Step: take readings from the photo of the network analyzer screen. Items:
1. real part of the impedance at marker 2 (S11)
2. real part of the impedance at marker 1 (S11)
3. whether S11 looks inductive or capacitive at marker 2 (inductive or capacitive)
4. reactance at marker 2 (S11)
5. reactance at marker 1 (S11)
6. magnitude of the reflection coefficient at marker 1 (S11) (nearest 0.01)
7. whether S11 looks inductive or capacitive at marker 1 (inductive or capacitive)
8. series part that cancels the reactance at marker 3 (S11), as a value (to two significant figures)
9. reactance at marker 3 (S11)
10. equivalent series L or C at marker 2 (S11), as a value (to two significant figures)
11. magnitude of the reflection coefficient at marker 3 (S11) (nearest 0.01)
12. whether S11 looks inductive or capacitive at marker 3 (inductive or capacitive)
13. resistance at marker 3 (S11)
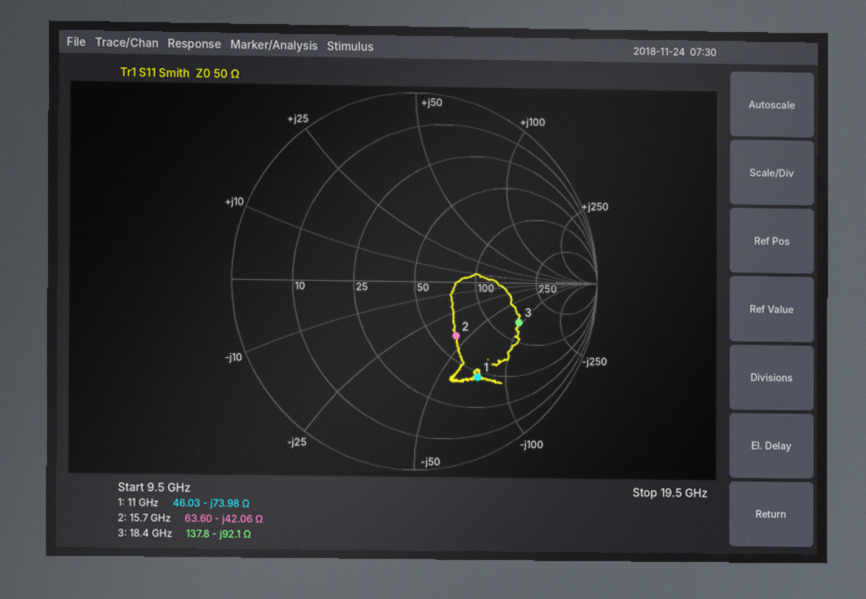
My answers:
63.60 Ω
46.03 Ω
capacitive
-42.06 Ω
-73.98 Ω
0.61
capacitive
800 pH
-92.1 Ω
240 fF
0.61
capacitive
137.8 Ω
